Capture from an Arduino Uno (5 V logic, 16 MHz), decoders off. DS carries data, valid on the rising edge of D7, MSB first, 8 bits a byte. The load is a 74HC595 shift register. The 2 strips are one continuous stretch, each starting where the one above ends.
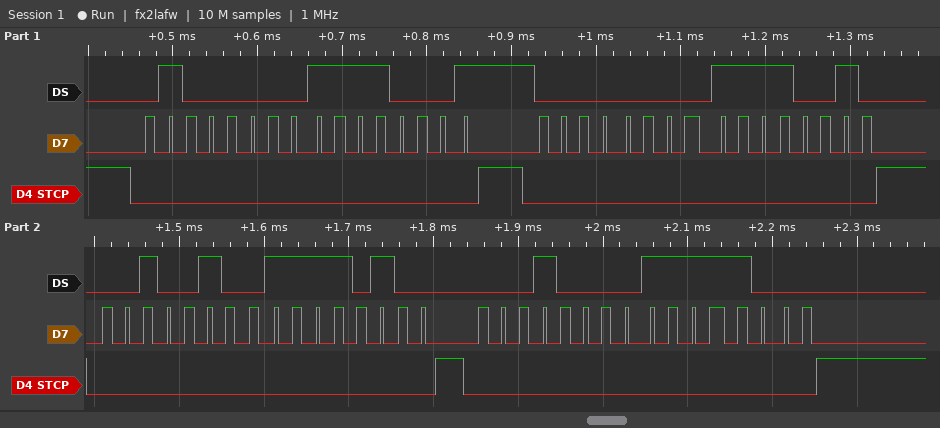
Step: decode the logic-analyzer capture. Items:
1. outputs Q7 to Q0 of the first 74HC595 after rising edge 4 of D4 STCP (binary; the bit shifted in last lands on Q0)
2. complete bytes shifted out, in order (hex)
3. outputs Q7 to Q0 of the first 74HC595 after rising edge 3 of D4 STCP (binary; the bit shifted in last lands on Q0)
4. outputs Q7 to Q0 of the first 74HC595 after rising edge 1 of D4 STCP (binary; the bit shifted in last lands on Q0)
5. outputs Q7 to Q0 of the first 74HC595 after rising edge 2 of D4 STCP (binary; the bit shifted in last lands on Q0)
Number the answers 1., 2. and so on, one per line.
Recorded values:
1. 11111000
2. 0x40 0xF1 0x00 0xF2 0x24 0xF4 0x10 0xF8
3. 11110100
4. 11110001
5. 11110010
